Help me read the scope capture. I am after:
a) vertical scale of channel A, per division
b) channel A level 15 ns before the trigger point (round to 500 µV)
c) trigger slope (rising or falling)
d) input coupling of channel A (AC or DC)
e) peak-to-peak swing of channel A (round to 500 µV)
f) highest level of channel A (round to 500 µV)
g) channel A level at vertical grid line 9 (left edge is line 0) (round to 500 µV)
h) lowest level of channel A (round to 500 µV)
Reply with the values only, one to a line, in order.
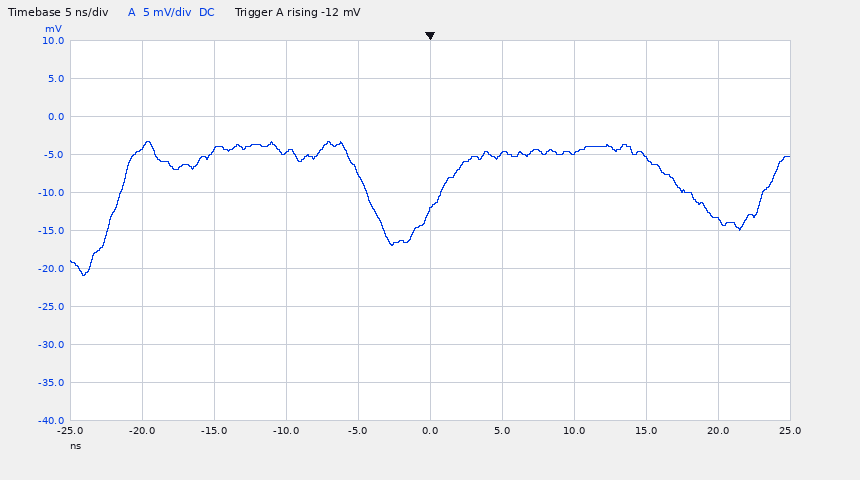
5 mV
-4.5 mV
rising
DC
17.5 mV
-3.5 mV
-13.5 mV
-21.0 mV
